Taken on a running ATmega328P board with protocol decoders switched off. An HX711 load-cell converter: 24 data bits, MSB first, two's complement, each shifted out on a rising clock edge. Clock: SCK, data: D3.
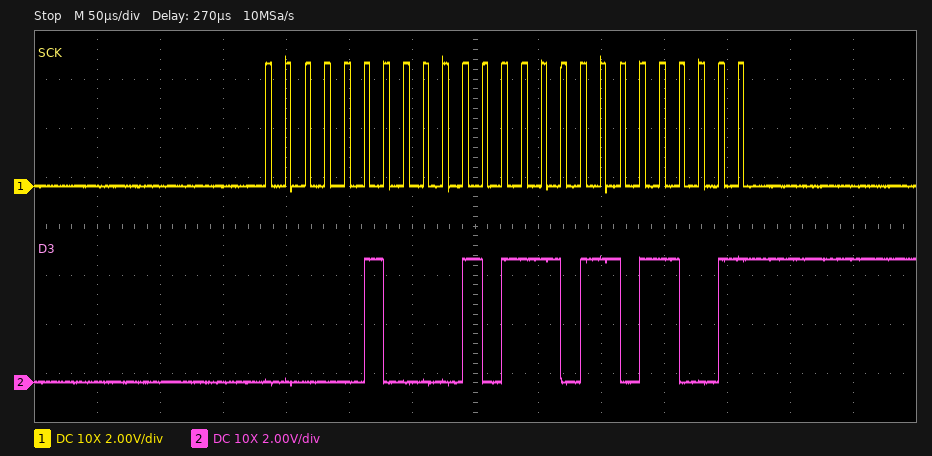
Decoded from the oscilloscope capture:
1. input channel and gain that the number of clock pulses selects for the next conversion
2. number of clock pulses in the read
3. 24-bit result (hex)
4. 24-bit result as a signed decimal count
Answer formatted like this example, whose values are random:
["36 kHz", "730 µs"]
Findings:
["channel A, gain 128", "25", "0x042ED9", "274137"]
